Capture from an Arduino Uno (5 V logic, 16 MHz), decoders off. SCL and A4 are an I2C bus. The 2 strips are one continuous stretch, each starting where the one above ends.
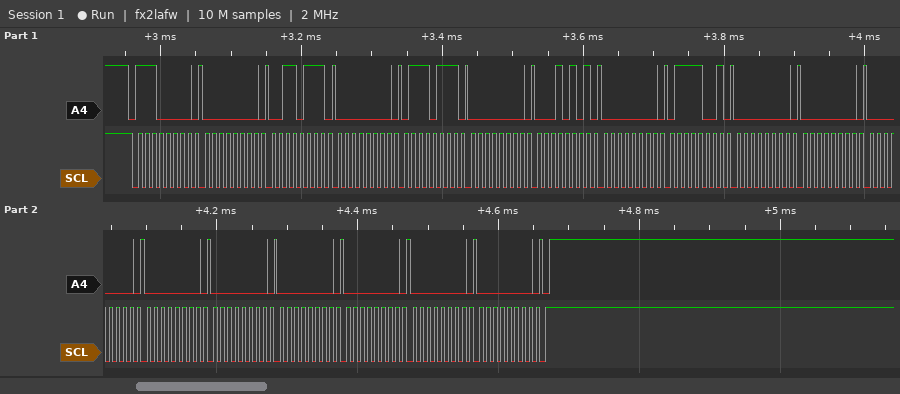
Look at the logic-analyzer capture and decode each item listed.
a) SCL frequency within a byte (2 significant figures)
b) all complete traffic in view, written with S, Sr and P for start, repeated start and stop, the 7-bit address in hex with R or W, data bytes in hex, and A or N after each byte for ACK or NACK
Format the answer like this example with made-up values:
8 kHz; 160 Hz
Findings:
100 kHz; S 70W A 00 A 37 A 00 A 77 A 00 A 15 A 00 A 79 A 00 A 00 A 00 A 00 A 00 A 00 A 00 A 00 A 00 A P
